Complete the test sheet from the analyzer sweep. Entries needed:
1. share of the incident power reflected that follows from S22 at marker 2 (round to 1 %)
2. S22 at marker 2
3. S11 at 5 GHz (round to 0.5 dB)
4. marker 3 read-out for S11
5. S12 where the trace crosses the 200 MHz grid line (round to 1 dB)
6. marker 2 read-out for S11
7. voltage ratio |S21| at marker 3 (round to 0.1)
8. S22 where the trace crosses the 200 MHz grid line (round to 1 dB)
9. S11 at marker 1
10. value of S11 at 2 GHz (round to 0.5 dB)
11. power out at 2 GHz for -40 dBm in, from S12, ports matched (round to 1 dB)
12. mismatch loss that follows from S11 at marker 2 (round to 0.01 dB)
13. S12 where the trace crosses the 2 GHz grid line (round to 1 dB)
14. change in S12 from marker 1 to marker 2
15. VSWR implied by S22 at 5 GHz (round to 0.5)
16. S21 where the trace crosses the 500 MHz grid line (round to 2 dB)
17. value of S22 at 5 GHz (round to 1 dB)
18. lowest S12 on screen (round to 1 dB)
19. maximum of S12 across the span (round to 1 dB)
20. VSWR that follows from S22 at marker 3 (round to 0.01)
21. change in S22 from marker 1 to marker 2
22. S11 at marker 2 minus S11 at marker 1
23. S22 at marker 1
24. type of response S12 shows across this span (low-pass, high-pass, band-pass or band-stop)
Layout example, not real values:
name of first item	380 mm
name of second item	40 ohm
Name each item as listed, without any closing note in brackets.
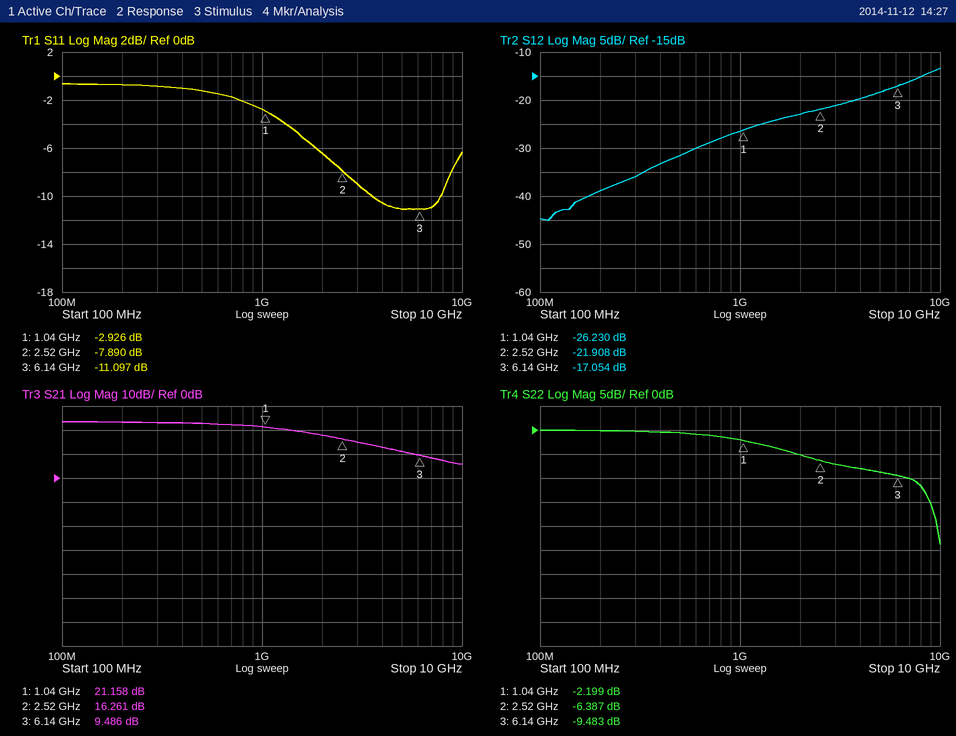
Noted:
share of the incident power reflected that follows from S22 at marker 2	23 %
S22 at marker 2	-6.387 dB
S11 at 5 GHz	-11.0 dB
marker 3 read-out for S11	-11.097 dB
S12 where the trace crosses the 200 MHz grid line	-39 dB
marker 2 read-out for S11	-7.890 dB
voltage ratio |S21| at marker 3	3.0
S22 where the trace crosses the 200 MHz grid line	0 dB
S11 at marker 1	-2.926 dB
value of S11 at 2 GHz	-6.5 dB
power out at 2 GHz for -40 dBm in, from S12, ports matched	-63 dBm
mismatch loss that follows from S11 at marker 2	0.77 dB
S12 where the trace crosses the 2 GHz grid line	-23 dB
change in S12 from marker 1 to marker 2	4.322 dB
VSWR implied by S22 at 5 GHz	2.0
S21 where the trace crosses the 500 MHz grid line	22 dB
value of S22 at 5 GHz	-9 dB
lowest S12 on screen	-45 dB
maximum of S12 across the span	-13 dB
VSWR that follows from S22 at marker 3	2.01
change in S22 from marker 1 to marker 2	-4.188 dB
S11 at marker 2 minus S11 at marker 1	-4.964 dB
S22 at marker 1	-2.199 dB
type of response S12 shows across this span	high-pass
